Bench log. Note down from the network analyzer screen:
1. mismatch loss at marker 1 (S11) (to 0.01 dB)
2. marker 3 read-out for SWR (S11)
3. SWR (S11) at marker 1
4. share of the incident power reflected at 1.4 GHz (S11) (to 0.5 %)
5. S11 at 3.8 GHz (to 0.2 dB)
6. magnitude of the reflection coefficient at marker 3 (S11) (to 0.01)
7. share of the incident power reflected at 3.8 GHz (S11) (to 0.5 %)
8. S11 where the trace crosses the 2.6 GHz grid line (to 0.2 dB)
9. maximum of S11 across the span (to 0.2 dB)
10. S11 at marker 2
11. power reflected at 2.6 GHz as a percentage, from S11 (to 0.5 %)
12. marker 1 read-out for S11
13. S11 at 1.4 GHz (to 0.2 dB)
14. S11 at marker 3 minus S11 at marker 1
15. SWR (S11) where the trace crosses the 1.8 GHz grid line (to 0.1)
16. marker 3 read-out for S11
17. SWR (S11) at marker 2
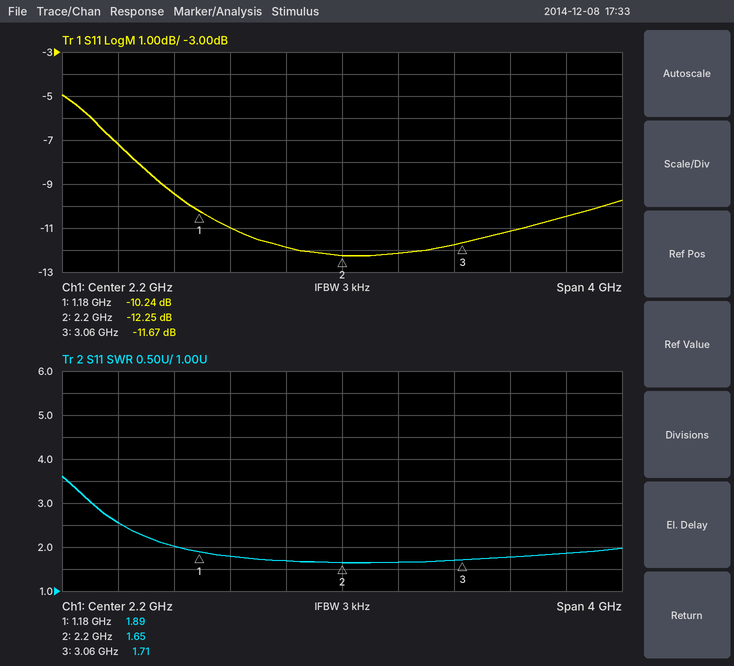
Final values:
0.43 dB
1.71
1.89
8.0 %
-10.4 dB
0.26
9.0 %
-12.2 dB
-5.0 dB
-12.25 dB
6.0 %
-10.24 dB
-11.0 dB
-1.43 dB
1.7
-11.67 dB
1.65
